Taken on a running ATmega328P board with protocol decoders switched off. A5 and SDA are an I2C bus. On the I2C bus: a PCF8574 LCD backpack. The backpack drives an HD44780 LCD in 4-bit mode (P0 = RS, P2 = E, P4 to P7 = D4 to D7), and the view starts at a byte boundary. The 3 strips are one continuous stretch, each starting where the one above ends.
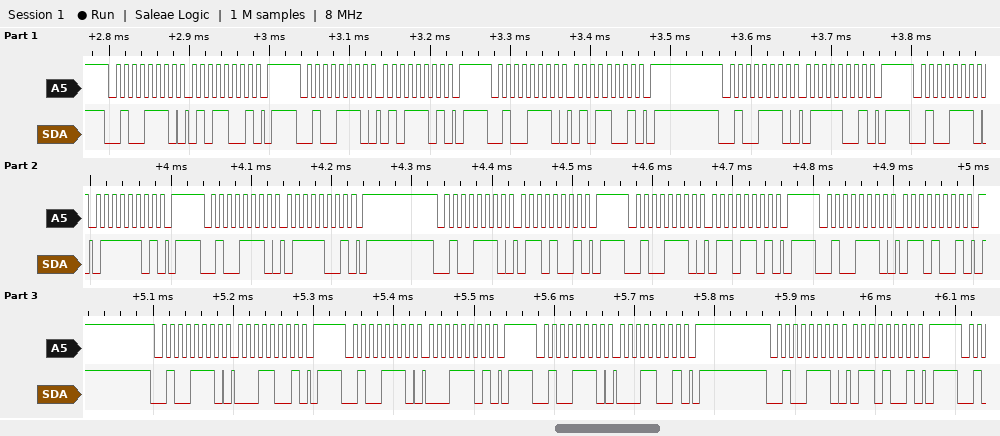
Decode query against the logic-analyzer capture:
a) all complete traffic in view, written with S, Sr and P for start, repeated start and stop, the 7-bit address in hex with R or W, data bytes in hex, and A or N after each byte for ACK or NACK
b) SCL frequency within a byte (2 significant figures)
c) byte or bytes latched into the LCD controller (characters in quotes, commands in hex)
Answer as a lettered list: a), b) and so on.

a) S 27W A 59 A P S 27W A 5D A P S 27W A 59 A P S 27W A 79 A P S 27W A 7D A P S 27W A 79 A P S 27W A 69 A P S 27W A 6D A P S 27W A 69 A P S 27W A 19 A P S 27W A 1D A P S 27W A 19 A P S 27W A 69 A P
b) 100 kHz
c) 'W' 'a'
